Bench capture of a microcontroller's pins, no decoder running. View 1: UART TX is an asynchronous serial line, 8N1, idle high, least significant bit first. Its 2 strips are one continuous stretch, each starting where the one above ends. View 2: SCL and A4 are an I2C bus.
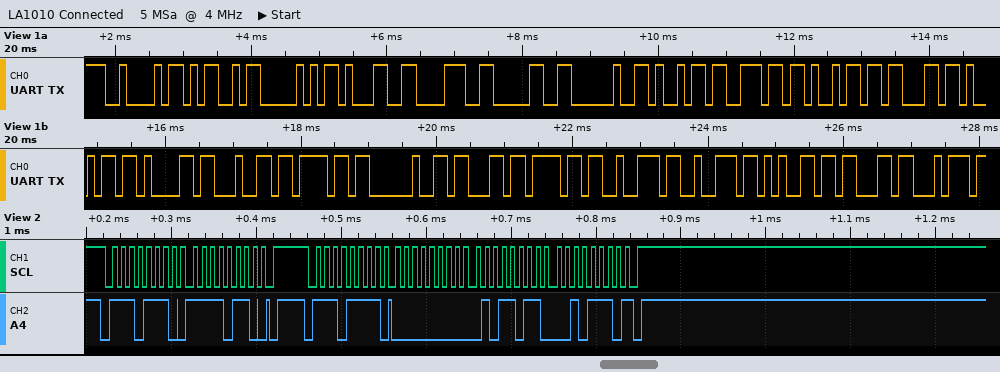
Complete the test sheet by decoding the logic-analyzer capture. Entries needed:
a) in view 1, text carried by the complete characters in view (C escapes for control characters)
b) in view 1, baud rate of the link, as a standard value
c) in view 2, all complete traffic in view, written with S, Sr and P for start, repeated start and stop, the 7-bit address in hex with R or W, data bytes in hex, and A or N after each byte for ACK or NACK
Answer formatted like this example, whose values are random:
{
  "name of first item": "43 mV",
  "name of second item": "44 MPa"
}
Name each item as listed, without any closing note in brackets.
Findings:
{
  "in view 1, text carried by the complete characters in view": "\"BMP180 iniciado correct\"",
  "in view 1, baud rate of the link, as a standard value": "9600 baud",
  "in view 2, all complete traffic in view, written with S, Sr and P for start, repeated start and stop, the 7-bit address in hex with R or W, data bytes in hex, and A or N after each byte for ACK or NACK": "S 77W A F6 A P S 77R A 00 A 5B A 2E N P"
}
